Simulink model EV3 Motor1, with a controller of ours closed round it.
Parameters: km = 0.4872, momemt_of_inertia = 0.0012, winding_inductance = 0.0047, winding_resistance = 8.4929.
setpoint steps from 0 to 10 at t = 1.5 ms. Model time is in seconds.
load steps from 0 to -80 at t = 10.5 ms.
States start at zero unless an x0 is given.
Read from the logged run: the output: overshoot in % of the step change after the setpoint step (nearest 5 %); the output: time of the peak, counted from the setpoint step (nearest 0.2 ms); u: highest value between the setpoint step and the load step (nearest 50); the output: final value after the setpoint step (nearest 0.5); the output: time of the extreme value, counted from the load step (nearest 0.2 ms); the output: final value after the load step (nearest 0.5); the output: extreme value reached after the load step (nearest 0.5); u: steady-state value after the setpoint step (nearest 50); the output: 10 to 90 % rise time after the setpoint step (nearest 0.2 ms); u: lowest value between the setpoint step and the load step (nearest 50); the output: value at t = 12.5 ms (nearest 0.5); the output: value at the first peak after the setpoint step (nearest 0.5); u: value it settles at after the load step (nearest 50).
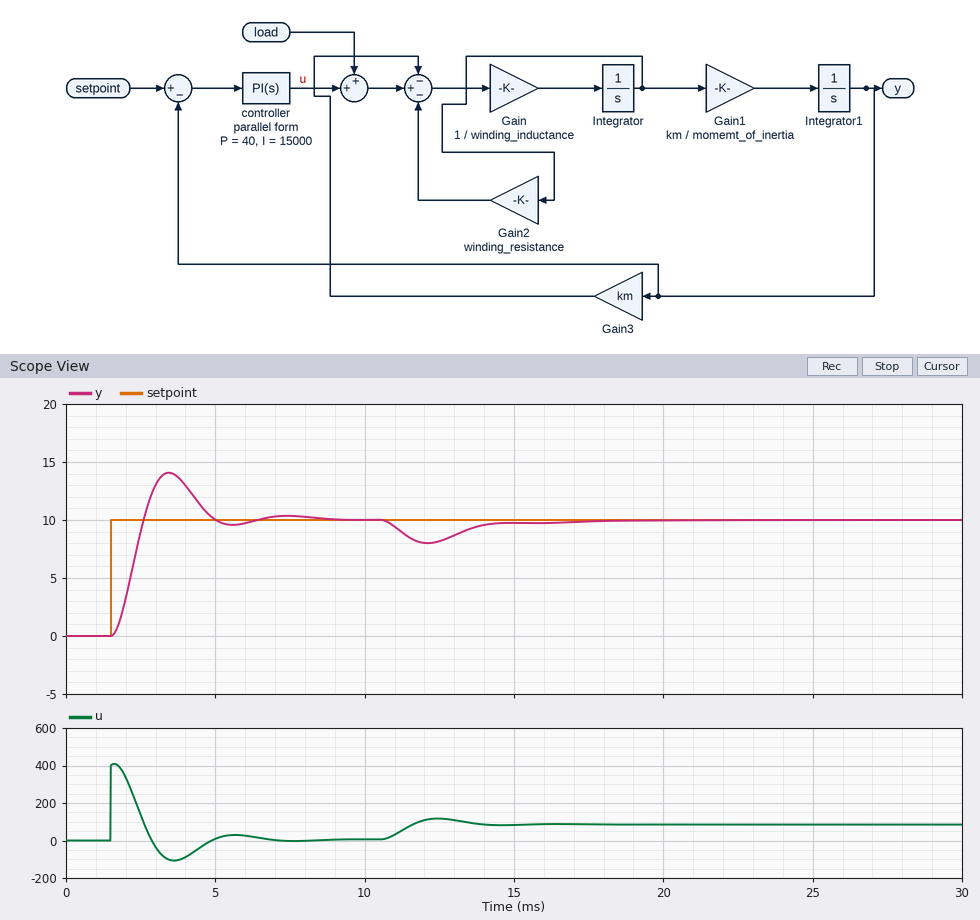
40 %
2.0 ms
400
10.0
1.6 ms
10.0
8.0
0
0.8 ms
-100
8.0
14.0
100
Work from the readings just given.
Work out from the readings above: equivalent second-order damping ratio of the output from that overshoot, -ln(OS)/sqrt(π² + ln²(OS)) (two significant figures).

0.28
